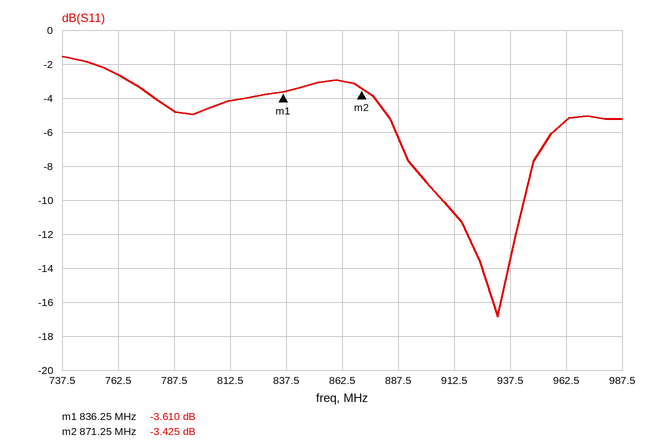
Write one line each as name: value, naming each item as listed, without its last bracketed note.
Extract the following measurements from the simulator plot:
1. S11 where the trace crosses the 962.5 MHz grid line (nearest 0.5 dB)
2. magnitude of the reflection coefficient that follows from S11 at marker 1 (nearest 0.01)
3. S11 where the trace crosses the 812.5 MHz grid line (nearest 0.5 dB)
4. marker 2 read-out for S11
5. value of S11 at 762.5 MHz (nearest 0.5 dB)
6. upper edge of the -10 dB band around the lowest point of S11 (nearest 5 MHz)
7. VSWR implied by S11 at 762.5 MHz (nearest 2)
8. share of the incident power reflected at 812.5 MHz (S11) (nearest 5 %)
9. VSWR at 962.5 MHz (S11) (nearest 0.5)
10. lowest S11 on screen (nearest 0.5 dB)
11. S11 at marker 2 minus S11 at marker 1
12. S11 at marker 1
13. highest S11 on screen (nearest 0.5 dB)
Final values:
S11 where the trace crosses the 962.5 MHz grid line: -5.5 dB
magnitude of the reflection coefficient that follows from S11 at marker 1: 0.66
S11 where the trace crosses the 812.5 MHz grid line: -4.0 dB
marker 2 read-out for S11: -3.425 dB
value of S11 at 762.5 MHz: -2.5 dB
upper edge of the -10 dB band around the lowest point of S11: 945 MHz
VSWR implied by S11 at 762.5 MHz: 6
share of the incident power reflected at 812.5 MHz (S11): 40 %
VSWR at 962.5 MHz (S11): 3.5
lowest S11 on screen: -17.0 dB
S11 at marker 2 minus S11 at marker 1: 0.185 dB
S11 at marker 1: -3.610 dB
highest S11 on screen: -1.5 dB
